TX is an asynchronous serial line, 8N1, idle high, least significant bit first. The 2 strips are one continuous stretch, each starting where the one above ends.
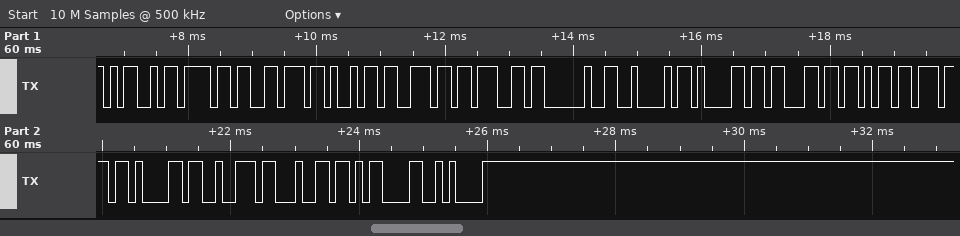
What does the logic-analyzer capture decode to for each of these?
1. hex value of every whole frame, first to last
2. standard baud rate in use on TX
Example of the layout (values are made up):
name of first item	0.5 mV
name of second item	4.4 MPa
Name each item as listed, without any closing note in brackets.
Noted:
hex value of every whole frame, first to last	4D 6F 76 69 6E 67 20 42 61 63 6B 77 61 72 64 0D 0A
standard baud rate in use on TX	9600 baud
